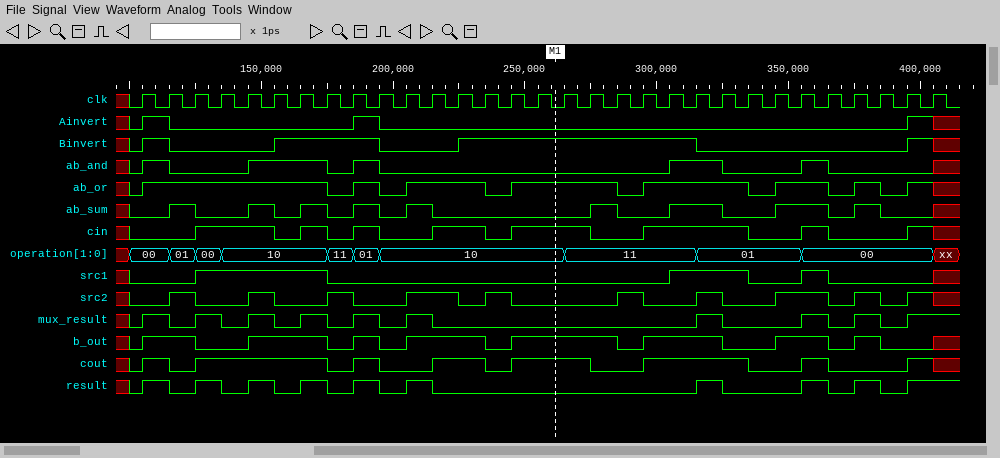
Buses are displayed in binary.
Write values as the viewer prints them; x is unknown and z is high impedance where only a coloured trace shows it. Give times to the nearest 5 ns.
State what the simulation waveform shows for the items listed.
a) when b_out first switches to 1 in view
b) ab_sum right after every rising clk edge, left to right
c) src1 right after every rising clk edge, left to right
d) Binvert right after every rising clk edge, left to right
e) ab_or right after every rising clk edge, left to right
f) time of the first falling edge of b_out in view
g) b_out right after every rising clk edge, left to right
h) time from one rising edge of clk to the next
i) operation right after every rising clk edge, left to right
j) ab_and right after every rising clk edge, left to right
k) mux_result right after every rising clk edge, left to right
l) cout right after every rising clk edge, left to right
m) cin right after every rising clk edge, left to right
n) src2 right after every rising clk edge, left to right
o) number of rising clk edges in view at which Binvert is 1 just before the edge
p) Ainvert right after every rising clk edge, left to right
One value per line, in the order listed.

105 ns
0 1 0 0 1 0 1 0 1 0 1 0 0 0 0 0 0 1 0 0 1 1 0 0 1 1 0 1 0 0 x
0 0 1 1 1 1 1 0 0 0 0 0 0 0 0 0 0 0 0 0 1 1 1 0 0 1 0 0 0 0 x
1 0 0 0 0 1 1 1 1 0 0 0 1 1 1 1 1 1 1 1 1 0 0 0 0 0 0 0 0 1 x
1 1 1 1 1 1 1 0 1 0 1 1 1 0 1 1 1 1 0 1 1 1 1 0 1 1 0 1 0 1 x
125 ns
1 1 0 0 1 1 1 0 1 0 1 1 1 0 1 1 1 1 0 1 1 1 0 0 1 1 0 1 0 0 x
10 ns
00, 01, 00, 10, 10, 10, 10, 11, 01, 10, 10, 10, 10, 10, 10, 10, 11, 11, 11, 11, 11, 01, 01, 01, 01, 00, 00, 00, 00, 00, xx
1 0 0 0 1 1 1 0 1 0 0 0 0 0 0 0 0 0 0 0 1 1 0 0 0 1 0 0 0 0 x
1 0 1 0 1 0 1 0 1 0 1 0 0 0 0 0 0 0 0 0 0 1 0 0 0 1 0 1 0 1 1
1 0 1 1 1 1 1 0 1 0 0 1 1 0 1 1 1 0 0 1 1 1 1 0 0 1 0 0 0 1 x
0 0 1 1 1 0 1 0 1 0 0 1 1 0 1 1 1 0 0 1 1 1 1 0 0 1 0 0 0 1 x
0 1 0 0 1 0 0 1 0 0 1 1 0 1 0 0 0 0 1 0 0 1 0 0 1 1 0 1 0 1 x
15
1 0 0 0 0 0 0 0 1 0 0 0 0 0 0 0 0 0 0 0 0 0 0 0 0 0 0 0 0 1 x
